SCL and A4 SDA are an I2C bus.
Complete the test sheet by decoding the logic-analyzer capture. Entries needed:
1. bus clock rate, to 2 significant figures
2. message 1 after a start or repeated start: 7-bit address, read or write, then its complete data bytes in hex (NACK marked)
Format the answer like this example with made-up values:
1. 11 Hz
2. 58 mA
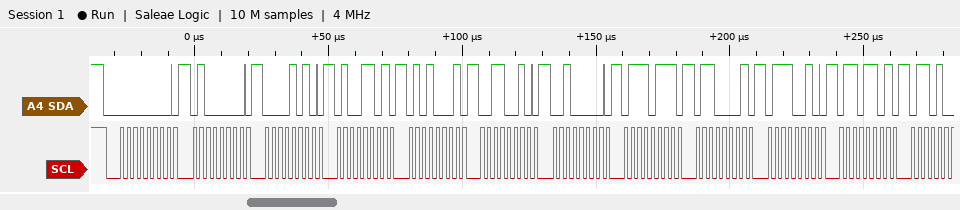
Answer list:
1. 400 kHz
2. 0x00 write: 40 0A 4D 51 32 20 77 61 72 6D
